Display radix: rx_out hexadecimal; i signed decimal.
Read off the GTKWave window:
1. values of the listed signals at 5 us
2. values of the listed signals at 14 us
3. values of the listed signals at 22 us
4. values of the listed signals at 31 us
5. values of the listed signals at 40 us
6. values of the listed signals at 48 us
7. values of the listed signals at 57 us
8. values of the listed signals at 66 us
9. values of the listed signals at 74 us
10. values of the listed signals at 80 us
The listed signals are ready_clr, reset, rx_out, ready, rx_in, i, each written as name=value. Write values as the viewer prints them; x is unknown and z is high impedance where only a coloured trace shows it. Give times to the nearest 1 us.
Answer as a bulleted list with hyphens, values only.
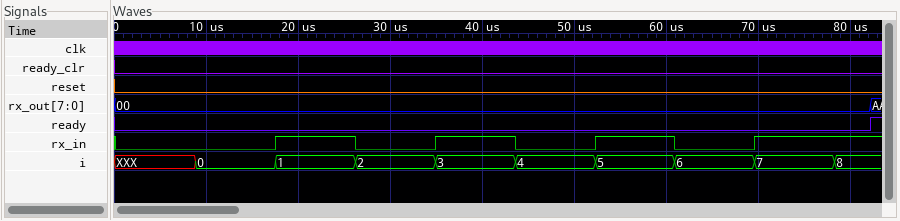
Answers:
- ready_clr=0, reset=0, rx_out=00, ready=0, rx_in=0, i=XXX
- ready_clr=0, reset=0, rx_out=00, ready=0, rx_in=0, i=0
- ready_clr=0, reset=0, rx_out=00, ready=0, rx_in=1, i=1
- ready_clr=0, reset=0, rx_out=00, ready=0, rx_in=0, i=2
- ready_clr=0, reset=0, rx_out=00, ready=0, rx_in=1, i=3
- ready_clr=0, reset=0, rx_out=00, ready=0, rx_in=0, i=4
- ready_clr=0, reset=0, rx_out=00, ready=0, rx_in=1, i=5
- ready_clr=0, reset=0, rx_out=00, ready=0, rx_in=0, i=6
- ready_clr=0, reset=0, rx_out=00, ready=0, rx_in=1, i=7
- ready_clr=0, reset=0, rx_out=00, ready=0, rx_in=1, i=8
